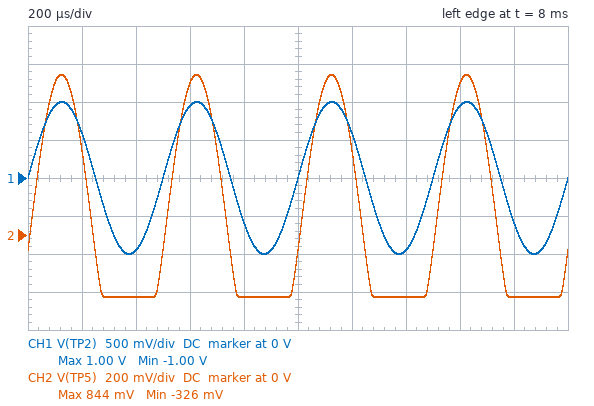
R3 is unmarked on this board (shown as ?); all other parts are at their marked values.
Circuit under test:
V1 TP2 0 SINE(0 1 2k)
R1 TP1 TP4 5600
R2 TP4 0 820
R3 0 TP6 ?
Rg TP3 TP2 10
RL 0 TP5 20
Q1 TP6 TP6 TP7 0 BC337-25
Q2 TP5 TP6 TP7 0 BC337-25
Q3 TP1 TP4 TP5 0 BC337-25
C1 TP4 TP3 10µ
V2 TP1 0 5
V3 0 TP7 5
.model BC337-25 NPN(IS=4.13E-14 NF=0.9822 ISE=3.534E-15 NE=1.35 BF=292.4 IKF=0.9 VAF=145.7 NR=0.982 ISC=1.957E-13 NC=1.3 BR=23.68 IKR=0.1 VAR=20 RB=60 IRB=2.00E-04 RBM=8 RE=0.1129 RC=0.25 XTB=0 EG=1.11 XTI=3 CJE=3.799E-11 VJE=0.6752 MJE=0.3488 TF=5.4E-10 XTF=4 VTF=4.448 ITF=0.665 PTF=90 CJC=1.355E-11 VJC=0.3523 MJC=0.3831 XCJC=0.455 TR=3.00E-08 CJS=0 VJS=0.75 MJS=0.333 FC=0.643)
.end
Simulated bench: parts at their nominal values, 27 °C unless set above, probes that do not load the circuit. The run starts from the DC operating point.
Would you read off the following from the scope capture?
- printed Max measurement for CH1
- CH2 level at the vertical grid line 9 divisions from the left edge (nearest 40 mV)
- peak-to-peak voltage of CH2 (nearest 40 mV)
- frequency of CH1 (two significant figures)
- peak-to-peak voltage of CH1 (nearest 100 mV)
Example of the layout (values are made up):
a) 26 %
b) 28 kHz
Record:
a) 1.00 V
b) -320 mV
c) 1.16 V
d) 2.0 kHz
e) 2.0 V
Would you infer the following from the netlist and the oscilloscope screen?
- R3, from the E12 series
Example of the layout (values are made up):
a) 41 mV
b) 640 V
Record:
a) 270 Ω
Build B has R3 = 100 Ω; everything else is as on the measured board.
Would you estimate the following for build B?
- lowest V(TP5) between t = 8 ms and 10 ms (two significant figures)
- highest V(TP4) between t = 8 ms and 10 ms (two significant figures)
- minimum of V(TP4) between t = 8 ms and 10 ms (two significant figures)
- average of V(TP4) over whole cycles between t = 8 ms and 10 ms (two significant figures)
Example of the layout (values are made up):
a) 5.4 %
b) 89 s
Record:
a) -870 mV
b) 1.5 V
c) -450 mV
d) 540 mV
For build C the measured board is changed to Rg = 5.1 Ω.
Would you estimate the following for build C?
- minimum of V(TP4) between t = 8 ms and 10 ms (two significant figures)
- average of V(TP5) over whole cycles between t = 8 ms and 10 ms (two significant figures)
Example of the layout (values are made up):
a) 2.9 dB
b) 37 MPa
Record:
a) -410 mV
b) 100 mV
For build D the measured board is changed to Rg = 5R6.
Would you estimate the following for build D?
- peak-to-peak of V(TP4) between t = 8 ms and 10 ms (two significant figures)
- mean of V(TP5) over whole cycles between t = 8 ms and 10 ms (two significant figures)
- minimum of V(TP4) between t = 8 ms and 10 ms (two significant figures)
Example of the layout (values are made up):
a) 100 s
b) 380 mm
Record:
a) 2.0 V
b) 100 mV
c) -410 mV
